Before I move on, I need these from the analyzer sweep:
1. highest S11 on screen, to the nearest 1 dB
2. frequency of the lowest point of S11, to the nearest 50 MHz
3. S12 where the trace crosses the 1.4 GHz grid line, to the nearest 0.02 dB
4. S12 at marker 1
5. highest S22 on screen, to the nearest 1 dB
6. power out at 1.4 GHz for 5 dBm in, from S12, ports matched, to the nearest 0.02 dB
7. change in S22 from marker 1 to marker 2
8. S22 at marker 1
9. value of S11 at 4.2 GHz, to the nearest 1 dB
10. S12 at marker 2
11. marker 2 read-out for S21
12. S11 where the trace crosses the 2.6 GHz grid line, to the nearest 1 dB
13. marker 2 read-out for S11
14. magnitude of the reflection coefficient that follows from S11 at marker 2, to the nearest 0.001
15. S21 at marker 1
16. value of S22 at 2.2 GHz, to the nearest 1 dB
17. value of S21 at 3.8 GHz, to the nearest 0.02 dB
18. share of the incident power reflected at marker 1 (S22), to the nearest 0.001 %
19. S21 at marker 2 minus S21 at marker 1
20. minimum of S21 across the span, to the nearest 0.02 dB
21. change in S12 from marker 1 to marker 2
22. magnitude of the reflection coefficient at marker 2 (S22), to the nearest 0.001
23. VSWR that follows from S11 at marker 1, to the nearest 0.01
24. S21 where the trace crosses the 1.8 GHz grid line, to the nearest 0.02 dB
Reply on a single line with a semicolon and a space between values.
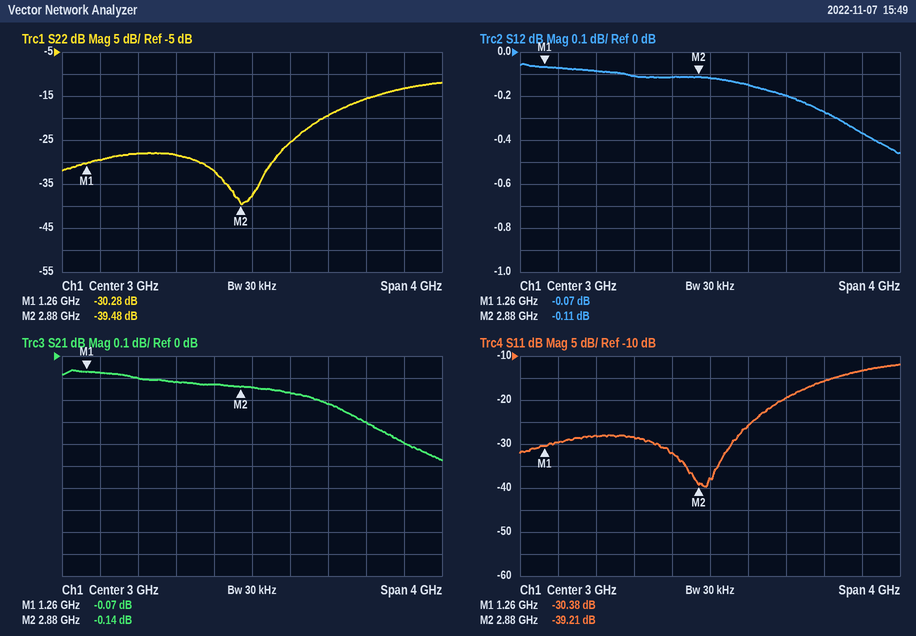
-12 dB; 2.95 GHz; -0.08 dB; -0.07 dB; -12 dB; 4.92 dBm; -9.20 dB; -30.28 dB; -16 dB; -0.11 dB; -0.14 dB; -32 dB; -39.21 dB; 0.011; -0.07 dB; -28 dB; -0.22 dB; 0.094 %; -0.07 dB; -0.48 dB; -0.04 dB; 0.011; 1.06; -0.10 dB
